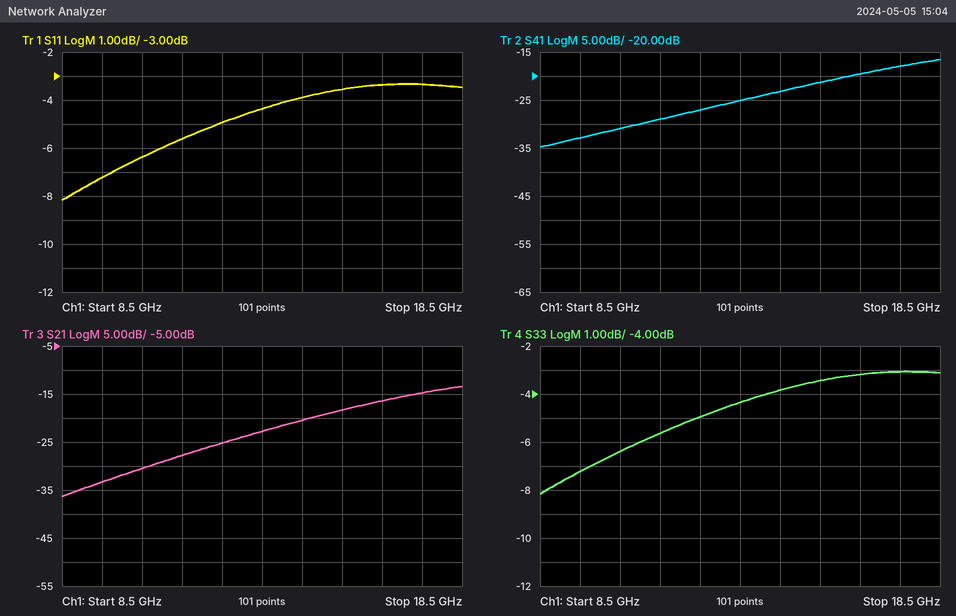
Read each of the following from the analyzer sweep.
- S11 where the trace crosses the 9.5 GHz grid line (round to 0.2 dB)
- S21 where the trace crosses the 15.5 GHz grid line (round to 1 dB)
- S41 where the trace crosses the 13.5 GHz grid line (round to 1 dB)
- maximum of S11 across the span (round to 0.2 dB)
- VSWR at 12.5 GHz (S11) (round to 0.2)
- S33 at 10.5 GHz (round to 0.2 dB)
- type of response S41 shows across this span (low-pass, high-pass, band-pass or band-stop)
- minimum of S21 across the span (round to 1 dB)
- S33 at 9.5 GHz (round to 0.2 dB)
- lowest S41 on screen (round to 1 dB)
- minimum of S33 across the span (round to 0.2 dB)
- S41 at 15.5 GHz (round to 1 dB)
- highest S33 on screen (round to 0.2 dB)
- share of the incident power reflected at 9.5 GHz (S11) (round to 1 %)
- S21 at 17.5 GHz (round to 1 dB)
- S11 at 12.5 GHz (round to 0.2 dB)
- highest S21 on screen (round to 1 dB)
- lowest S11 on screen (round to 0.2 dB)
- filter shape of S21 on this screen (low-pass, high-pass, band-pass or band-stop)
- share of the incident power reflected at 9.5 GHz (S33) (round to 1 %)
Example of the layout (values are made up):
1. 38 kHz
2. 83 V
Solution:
1. -7.2 dB
2. -18 dB
3. -25 dB
4. -3.4 dB
5. 3.6
6. -6.4 dB
7. high-pass
8. -36 dB
9. -7.2 dB
10. -35 dB
11. -8.2 dB
12. -21 dB
13. -3.0 dB
14. 19 %
15. -15 dB
16. -5.0 dB
17. -13 dB
18. -8.2 dB
19. high-pass
20. 19 %
